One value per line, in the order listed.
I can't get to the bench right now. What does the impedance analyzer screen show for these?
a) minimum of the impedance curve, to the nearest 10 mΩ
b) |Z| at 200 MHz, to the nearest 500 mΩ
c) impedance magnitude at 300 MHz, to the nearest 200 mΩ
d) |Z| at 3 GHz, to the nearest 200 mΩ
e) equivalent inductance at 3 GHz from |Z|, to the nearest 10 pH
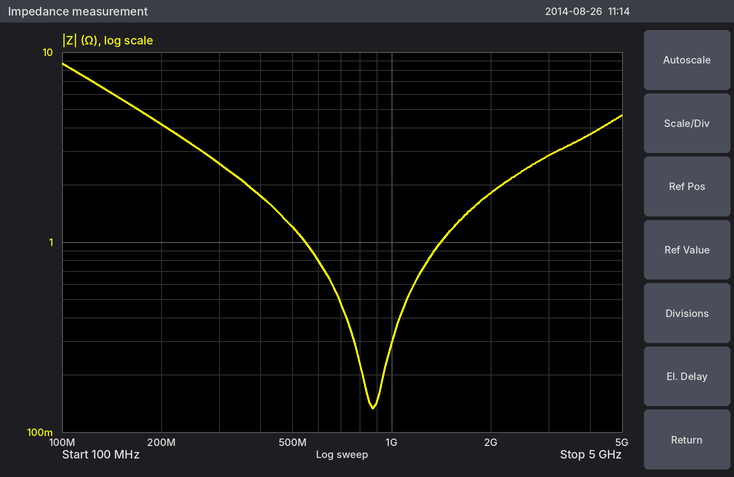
130 mΩ
4.0 Ω
2.6 Ω
2.8 Ω
150 pH
